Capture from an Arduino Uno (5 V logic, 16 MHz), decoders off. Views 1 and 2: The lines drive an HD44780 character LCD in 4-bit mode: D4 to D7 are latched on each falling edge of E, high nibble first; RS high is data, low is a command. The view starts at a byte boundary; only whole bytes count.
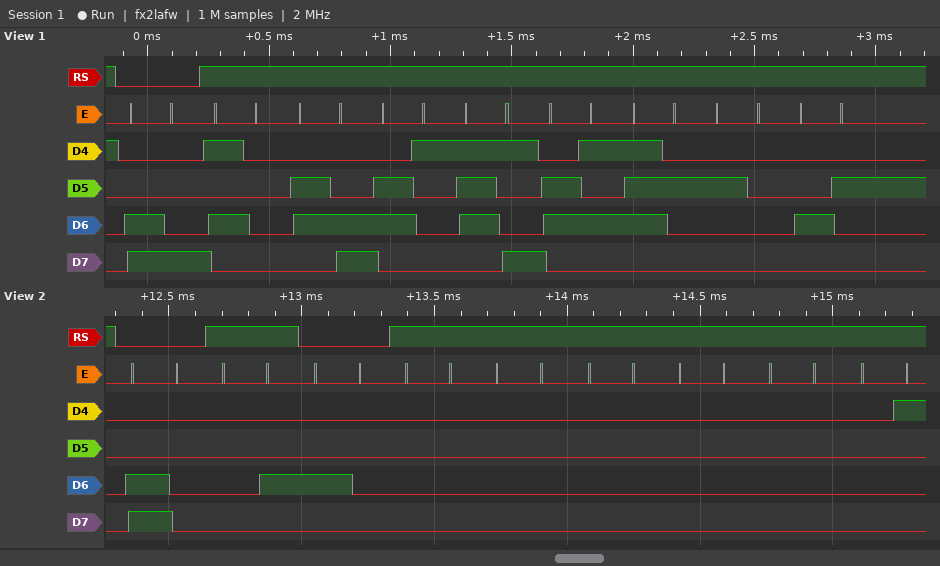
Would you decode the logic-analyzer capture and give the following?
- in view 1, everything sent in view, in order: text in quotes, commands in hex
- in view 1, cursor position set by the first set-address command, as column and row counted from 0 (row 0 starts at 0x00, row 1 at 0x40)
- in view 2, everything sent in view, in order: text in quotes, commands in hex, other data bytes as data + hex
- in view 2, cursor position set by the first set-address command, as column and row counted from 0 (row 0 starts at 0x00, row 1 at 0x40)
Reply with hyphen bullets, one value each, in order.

- 0xC8 "Player B"
- column 8, row 1
- 0xC0 data 04 0x40 data 00 00 00 00 00 01
- column 0, row 1
